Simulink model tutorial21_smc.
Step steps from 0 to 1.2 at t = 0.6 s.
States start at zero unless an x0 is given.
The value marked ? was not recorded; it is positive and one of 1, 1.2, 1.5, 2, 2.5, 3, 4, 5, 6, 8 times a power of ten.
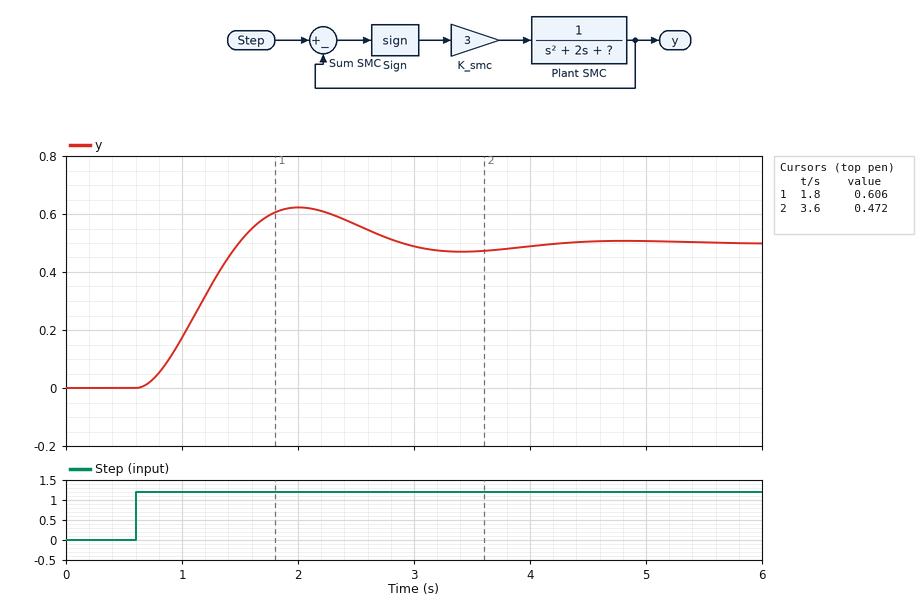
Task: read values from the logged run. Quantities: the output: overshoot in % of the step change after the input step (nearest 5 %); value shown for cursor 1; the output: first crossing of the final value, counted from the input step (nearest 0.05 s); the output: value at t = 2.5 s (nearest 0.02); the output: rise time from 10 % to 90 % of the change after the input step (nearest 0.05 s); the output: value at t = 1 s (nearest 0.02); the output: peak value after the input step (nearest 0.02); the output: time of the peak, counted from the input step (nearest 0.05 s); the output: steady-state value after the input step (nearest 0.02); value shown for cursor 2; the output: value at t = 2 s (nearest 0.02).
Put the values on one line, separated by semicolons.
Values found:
25 %; 0.606; 0.90 s; 0.56; 0.60 s; 0.18; 0.62; 1.40 s; 0.50; 0.472; 0.62
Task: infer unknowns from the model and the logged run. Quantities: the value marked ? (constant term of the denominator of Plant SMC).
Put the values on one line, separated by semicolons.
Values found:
6
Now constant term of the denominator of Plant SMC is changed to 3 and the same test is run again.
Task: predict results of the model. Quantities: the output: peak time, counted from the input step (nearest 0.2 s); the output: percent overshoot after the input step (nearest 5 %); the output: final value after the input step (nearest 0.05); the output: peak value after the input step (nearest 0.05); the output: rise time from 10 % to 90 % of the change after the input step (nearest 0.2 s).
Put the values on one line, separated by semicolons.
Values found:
2.2 s; 10 %; 1.00; 1.10; 1.0 s
